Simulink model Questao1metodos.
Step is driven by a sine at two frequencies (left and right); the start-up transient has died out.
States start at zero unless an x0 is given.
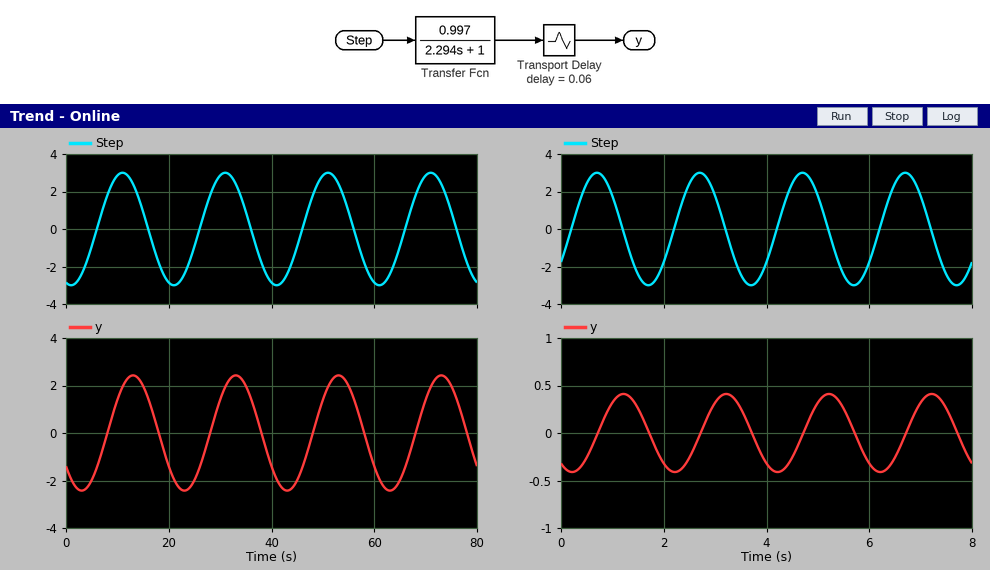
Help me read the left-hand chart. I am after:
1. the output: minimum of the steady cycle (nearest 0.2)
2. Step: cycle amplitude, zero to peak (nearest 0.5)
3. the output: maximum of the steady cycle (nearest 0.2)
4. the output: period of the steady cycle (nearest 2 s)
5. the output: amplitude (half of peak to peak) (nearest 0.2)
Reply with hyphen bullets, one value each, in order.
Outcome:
- -2.4
- 3.0
- 2.4
- 20 s
- 2.4
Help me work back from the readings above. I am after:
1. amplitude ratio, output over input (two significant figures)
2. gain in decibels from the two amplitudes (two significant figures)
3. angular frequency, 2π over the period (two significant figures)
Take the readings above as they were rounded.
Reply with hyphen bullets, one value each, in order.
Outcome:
- 0.80
- -1.9 dB
- 0.31 rad/s
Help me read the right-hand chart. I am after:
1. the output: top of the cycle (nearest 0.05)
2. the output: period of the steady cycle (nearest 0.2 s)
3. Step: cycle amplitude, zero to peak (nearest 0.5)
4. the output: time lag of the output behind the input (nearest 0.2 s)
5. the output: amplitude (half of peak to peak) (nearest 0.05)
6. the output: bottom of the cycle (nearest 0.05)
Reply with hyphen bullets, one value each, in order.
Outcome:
- 0.40
- 2.0 s
- 3.0
- 0.6 s
- 0.40
- -0.40
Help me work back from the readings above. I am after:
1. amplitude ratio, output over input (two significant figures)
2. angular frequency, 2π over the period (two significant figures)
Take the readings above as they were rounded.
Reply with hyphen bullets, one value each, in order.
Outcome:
- 0.13
- 3.1 rad/s
